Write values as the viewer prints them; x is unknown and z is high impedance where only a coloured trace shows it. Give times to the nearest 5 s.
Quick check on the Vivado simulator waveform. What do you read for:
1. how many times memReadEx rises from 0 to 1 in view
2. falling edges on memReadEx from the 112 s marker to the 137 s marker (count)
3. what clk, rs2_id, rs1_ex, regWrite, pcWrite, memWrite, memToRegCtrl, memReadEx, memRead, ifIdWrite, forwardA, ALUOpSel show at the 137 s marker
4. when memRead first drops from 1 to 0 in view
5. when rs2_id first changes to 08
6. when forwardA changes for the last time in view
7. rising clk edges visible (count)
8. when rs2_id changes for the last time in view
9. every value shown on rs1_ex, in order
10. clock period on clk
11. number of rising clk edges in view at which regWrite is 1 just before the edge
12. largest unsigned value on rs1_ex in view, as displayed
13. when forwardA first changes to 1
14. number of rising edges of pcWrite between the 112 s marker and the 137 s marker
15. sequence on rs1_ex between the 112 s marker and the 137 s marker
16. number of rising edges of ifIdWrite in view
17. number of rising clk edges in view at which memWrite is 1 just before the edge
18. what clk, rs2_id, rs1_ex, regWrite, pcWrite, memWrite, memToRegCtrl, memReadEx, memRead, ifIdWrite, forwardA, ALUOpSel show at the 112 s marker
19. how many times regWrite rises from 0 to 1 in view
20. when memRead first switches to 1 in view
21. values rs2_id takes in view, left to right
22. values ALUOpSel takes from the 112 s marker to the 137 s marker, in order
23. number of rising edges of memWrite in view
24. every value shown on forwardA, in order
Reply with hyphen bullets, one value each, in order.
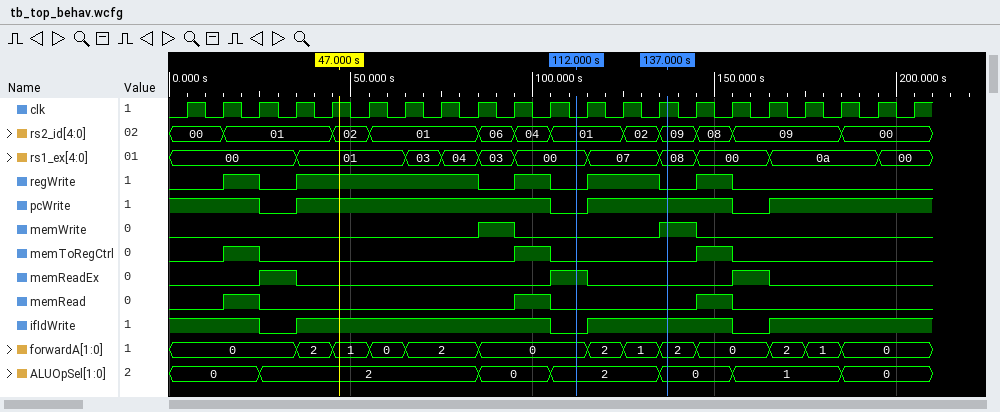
- 3
- 1
- clk=1, rs2_id=09, rs1_ex=08, regWrite=0, pcWrite=1, memWrite=1, memToRegCtrl=0, memReadEx=0, memRead=0, ifIdWrite=1, forwardA=2, ALUOpSel=0
- 25 s
- 145 s
- 185 s
- 21
- 185 s
- 00, 01, 03, 04, 03, 00, 07, 08, 00, 0a, 00
- 10 s
- 10
- 0a
- 45 s
- 1
- 00, 07, 08
- 3
- 2
- clk=0, rs2_id=01, rs1_ex=00, regWrite=0, pcWrite=0, memWrite=0, memToRegCtrl=0, memReadEx=1, memRead=0, ifIdWrite=0, forwardA=0, ALUOpSel=2
- 5
- 15 s
- 00, 01, 02, 01, 06, 04, 01, 02, 09, 08, 09, 00
- 2, 0
- 2
- 0, 2, 1, 0, 2, 0, 2, 1, 2, 0, 2, 1, 0
